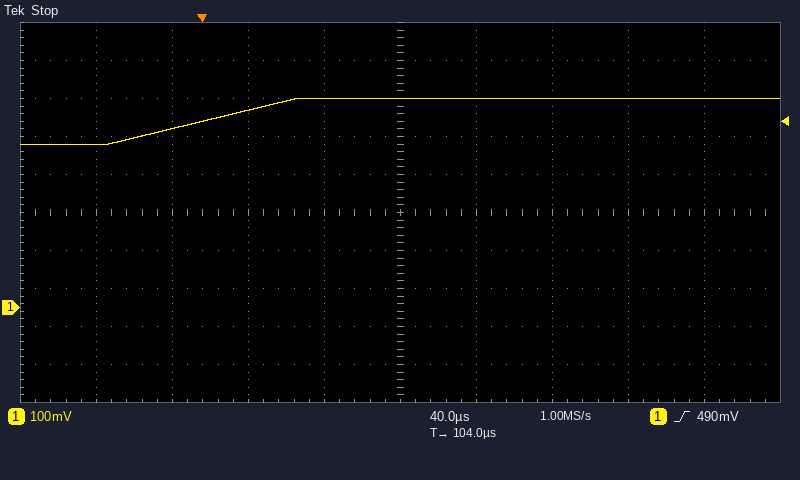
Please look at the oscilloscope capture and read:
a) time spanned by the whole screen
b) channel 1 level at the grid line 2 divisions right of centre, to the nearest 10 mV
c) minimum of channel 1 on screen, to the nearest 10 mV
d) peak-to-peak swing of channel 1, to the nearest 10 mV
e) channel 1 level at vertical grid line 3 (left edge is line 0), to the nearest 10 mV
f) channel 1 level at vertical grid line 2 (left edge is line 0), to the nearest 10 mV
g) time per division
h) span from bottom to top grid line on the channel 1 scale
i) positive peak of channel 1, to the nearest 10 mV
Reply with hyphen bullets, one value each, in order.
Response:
- 400 µs
- 550 mV
- 430 mV
- 120 mV
- 520 mV
- 470 mV
- 40 µs
- 1 V
- 550 mV
